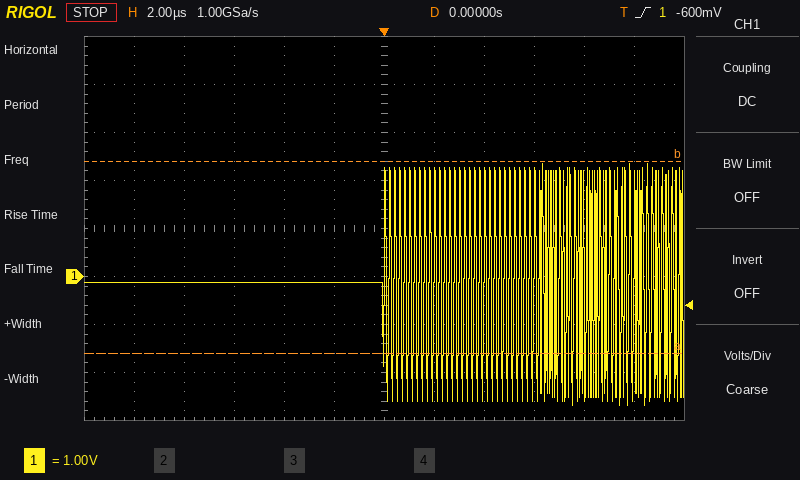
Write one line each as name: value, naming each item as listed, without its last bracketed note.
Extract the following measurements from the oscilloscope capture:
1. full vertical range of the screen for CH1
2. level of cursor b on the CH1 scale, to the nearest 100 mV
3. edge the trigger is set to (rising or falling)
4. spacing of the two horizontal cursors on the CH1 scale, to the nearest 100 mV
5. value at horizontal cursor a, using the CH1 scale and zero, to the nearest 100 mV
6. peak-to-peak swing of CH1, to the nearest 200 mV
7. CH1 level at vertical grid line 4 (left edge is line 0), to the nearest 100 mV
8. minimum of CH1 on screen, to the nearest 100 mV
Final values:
full vertical range of the screen for CH1: 8 V
level of cursor b on the CH1 scale, to the nearest 100 mV: 2.4 V
edge the trigger is set to: rising
spacing of the two horizontal cursors on the CH1 scale, to the nearest 100 mV: 4.0 V
value at horizontal cursor a, using the CH1 scale and zero, to the nearest 100 mV: -1.6 V
peak-to-peak swing of CH1, to the nearest 200 mV: 5.0 V
CH1 level at vertical grid line 4 (left edge is line 0), to the nearest 100 mV: -100 mV
minimum of CH1 on screen, to the nearest 100 mV: -2.7 V
